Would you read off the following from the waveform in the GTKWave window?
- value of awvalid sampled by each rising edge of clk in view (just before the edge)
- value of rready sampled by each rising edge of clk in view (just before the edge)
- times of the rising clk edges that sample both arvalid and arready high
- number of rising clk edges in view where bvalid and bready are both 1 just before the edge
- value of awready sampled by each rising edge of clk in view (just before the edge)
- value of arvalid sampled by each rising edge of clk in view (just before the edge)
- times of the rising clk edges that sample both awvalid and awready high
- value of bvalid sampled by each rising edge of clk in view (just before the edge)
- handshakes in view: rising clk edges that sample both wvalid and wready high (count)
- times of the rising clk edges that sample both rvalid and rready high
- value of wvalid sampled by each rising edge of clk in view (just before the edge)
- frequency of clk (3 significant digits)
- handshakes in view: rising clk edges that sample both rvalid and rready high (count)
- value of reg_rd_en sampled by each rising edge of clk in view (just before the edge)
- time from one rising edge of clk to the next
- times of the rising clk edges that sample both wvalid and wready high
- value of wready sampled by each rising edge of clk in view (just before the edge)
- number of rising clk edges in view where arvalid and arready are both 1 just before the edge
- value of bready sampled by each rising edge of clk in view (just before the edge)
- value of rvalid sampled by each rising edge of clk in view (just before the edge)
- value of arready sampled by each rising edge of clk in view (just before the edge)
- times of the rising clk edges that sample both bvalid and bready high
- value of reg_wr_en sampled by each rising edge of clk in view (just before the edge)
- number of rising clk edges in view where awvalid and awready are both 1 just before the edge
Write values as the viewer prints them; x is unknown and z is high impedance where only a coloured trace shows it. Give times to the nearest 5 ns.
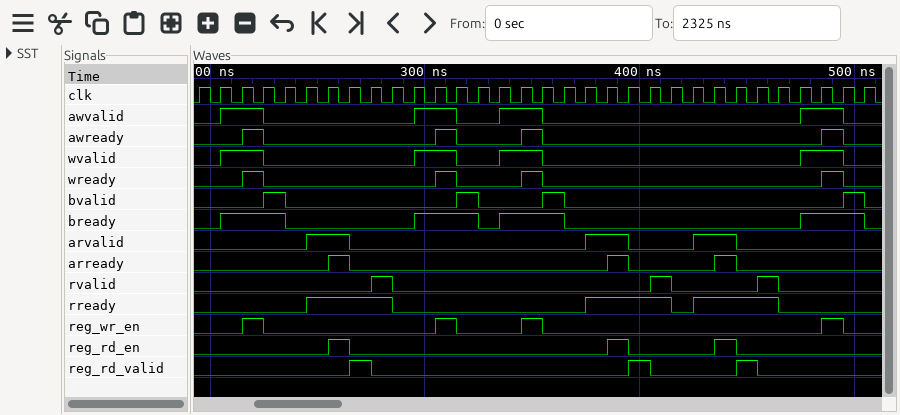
0 0 1 1 0 0 0 0 0 0 0 1 1 0 0 1 1 0 0 0 0 0 0 0 0 0 0 0 0 1 1 0
0 0 0 0 0 0 1 1 1 1 0 0 0 0 0 0 0 0 0 1 1 1 1 0 1 1 1 1 0 0 0 0
265 ns, 395 ns, 445 ns
4
0 0 0 1 0 0 0 0 0 0 0 0 1 0 0 0 1 0 0 0 0 0 0 0 0 0 0 0 0 0 1 0
0 0 0 0 0 0 1 1 0 0 0 0 0 0 0 0 0 0 0 1 1 0 0 0 1 1 0 0 0 0 0 0
225 ns, 315 ns, 355 ns, 495 ns
0 0 0 0 1 0 0 0 0 0 0 0 0 1 0 0 0 1 0 0 0 0 0 0 0 0 0 0 0 0 0 1
4
285 ns, 415 ns, 465 ns
0 0 1 1 0 0 0 0 0 0 0 1 1 0 0 1 1 0 0 0 0 0 0 0 0 0 0 0 0 1 1 0
100 MHz
3
0 0 0 0 0 0 0 1 0 0 0 0 0 0 0 0 0 0 0 0 1 0 0 0 0 1 0 0 0 0 0 0
10 ns
225 ns, 315 ns, 355 ns, 495 ns
0 0 0 1 0 0 0 0 0 0 0 0 1 0 0 0 1 0 0 0 0 0 0 0 0 0 0 0 0 0 1 0
3
0 0 1 1 1 0 0 0 0 0 0 1 1 1 0 1 1 1 0 0 0 0 0 0 0 0 0 0 0 1 1 1
0 0 0 0 0 0 0 0 0 1 0 0 0 0 0 0 0 0 0 0 0 0 1 0 0 0 0 1 0 0 0 0
0 0 0 0 0 0 0 1 0 0 0 0 0 0 0 0 0 0 0 0 1 0 0 0 0 1 0 0 0 0 0 0
235 ns, 325 ns, 365 ns, 505 ns
0 0 0 1 0 0 0 0 0 0 0 0 1 0 0 0 1 0 0 0 0 0 0 0 0 0 0 0 0 0 1 0
4
